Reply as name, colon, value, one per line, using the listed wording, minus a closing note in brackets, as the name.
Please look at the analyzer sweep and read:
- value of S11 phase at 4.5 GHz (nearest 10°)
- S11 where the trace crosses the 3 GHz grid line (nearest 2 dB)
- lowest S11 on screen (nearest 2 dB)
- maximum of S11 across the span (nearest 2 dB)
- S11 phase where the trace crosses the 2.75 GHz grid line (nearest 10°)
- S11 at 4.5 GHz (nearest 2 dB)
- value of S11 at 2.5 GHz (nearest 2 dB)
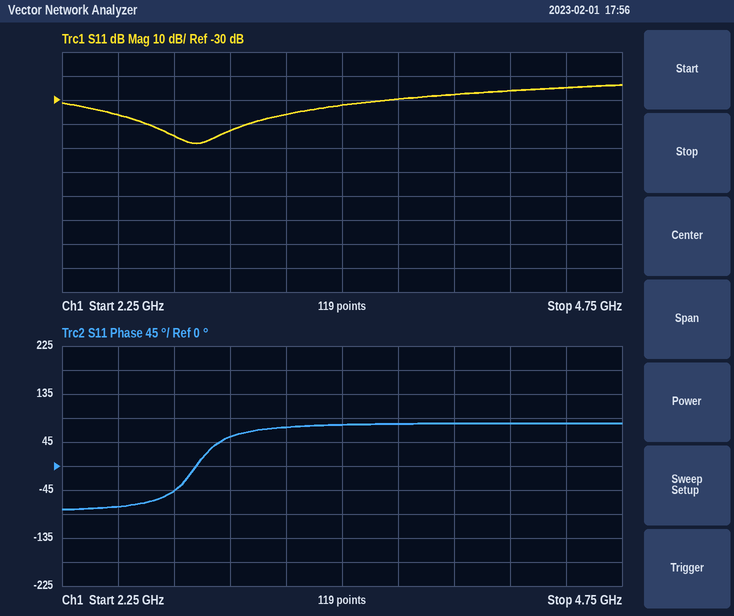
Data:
value of S11 phase at 4.5 GHz: 80°
S11 where the trace crosses the 3 GHz grid line: -42 dB
lowest S11 on screen: -48 dB
maximum of S11 across the span: -24 dB
S11 phase where the trace crosses the 2.75 GHz grid line: -50°
S11 at 4.5 GHz: -24 dB
value of S11 at 2.5 GHz: -36 dB
